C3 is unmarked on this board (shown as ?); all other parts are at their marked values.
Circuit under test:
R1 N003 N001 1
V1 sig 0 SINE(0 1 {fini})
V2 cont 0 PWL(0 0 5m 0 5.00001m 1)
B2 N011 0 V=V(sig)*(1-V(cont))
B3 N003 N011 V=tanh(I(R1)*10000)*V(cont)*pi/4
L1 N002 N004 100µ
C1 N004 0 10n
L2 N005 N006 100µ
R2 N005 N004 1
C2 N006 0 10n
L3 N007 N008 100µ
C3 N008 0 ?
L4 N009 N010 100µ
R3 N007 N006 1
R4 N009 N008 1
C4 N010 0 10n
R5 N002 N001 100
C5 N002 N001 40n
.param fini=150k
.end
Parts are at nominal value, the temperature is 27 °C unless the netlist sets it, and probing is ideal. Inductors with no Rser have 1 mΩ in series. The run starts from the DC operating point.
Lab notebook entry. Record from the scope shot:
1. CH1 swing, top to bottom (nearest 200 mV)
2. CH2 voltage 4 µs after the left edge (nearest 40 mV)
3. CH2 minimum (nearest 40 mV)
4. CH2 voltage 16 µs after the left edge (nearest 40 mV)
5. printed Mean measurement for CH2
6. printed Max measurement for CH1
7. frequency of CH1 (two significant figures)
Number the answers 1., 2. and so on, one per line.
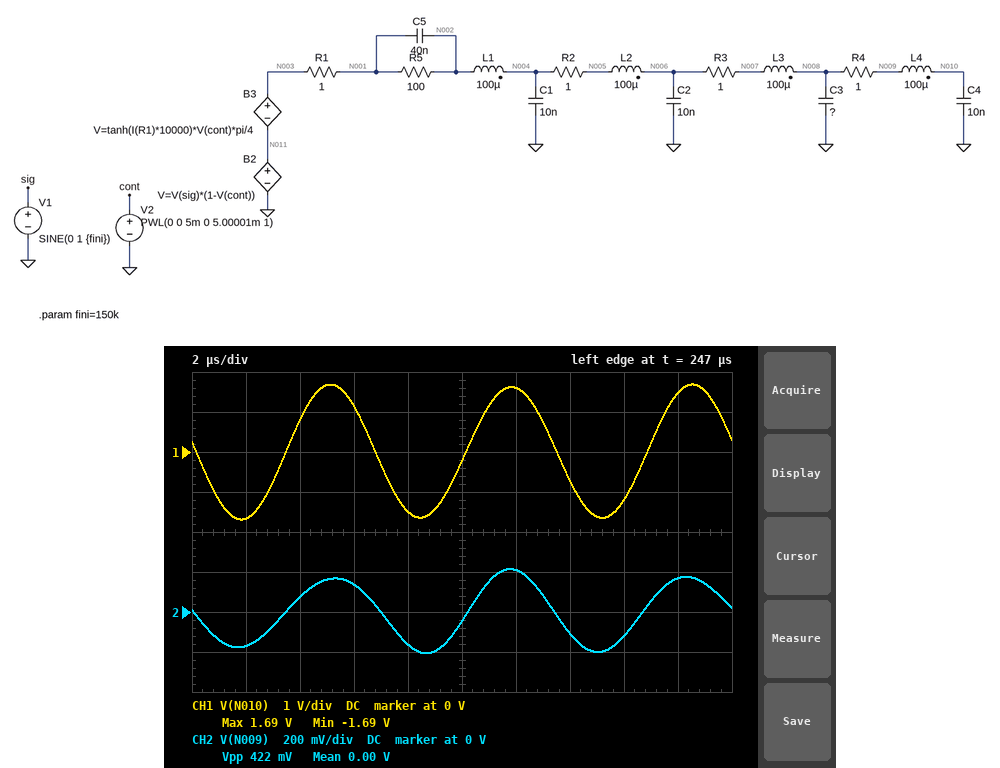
1. 3.4 V
2. 80 mV
3. -200 mV
4. -120 mV
5. 0.00 V
6. 1.69 V
7. 150 kHz
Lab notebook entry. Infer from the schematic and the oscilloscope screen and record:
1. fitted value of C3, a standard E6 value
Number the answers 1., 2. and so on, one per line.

1. 22 nF
